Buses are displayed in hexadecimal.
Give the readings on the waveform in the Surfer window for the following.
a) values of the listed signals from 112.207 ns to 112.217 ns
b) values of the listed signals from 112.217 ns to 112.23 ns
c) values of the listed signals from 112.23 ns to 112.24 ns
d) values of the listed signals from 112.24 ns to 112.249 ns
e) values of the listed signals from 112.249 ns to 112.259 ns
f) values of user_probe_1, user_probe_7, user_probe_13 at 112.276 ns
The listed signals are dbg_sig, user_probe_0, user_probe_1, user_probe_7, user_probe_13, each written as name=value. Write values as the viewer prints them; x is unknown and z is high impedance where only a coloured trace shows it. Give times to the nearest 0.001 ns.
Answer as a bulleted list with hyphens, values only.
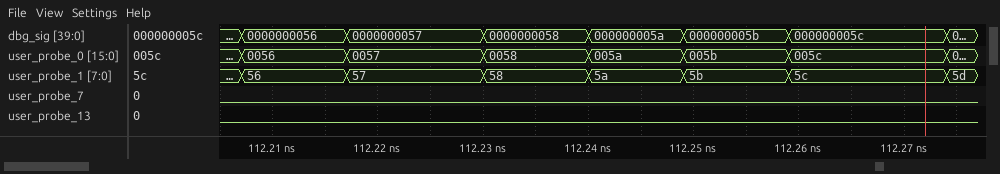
- dbg_sig=0000000056, user_probe_0=0056, user_probe_1=56, user_probe_7=0, user_probe_13=0
- dbg_sig=0000000057, user_probe_0=0057, user_probe_1=57, user_probe_7=0, user_probe_13=0
- dbg_sig=0000000058, user_probe_0=0058, user_probe_1=58, user_probe_7=0, user_probe_13=0
- dbg_sig=000000005a, user_probe_0=005a, user_probe_1=5a, user_probe_7=0, user_probe_13=0
- dbg_sig=000000005b, user_probe_0=005b, user_probe_1=5b, user_probe_7=0, user_probe_13=0
- user_probe_1=5d, user_probe_7=0, user_probe_13=0
